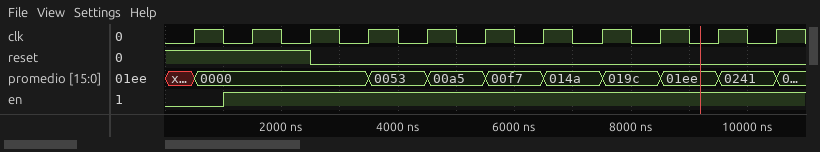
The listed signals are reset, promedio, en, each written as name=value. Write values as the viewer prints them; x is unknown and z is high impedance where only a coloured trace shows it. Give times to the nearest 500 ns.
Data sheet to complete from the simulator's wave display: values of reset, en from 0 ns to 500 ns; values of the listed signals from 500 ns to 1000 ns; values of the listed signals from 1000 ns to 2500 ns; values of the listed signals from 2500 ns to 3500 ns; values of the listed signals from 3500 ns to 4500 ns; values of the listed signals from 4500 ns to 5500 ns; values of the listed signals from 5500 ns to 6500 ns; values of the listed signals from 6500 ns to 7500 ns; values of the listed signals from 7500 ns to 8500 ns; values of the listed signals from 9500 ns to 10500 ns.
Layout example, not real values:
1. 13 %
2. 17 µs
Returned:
1. reset=1, en=0
2. reset=1, promedio=0000, en=0
3. reset=1, promedio=0000, en=1
4. reset=0, promedio=0000, en=1
5. reset=0, promedio=0053, en=1
6. reset=0, promedio=00a5, en=1
7. reset=0, promedio=00f7, en=1
8. reset=0, promedio=014a, en=1
9. reset=0, promedio=019c, en=1
10. reset=0, promedio=0241, en=1
